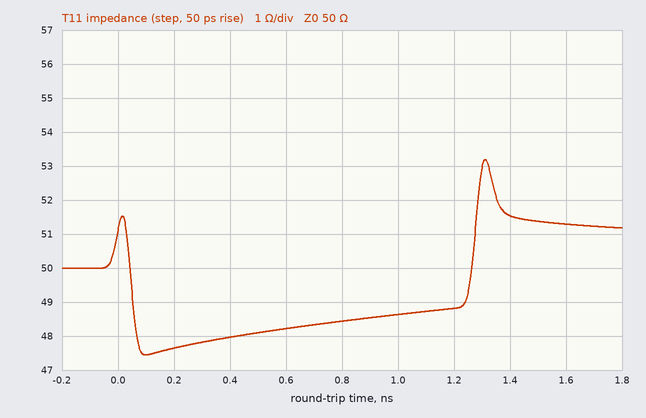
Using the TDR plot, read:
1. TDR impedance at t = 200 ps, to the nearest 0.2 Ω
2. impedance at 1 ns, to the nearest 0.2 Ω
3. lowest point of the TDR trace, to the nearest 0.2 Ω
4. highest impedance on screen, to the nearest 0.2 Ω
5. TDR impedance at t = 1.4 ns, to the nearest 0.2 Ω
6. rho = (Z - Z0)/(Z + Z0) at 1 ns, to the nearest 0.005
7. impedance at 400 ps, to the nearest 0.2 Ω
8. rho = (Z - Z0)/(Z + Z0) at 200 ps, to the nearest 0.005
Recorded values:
47.6 Ω
48.6 Ω
47.4 Ω
53.2 Ω
51.6 Ω
-0.015
48.0 Ω
-0.025
